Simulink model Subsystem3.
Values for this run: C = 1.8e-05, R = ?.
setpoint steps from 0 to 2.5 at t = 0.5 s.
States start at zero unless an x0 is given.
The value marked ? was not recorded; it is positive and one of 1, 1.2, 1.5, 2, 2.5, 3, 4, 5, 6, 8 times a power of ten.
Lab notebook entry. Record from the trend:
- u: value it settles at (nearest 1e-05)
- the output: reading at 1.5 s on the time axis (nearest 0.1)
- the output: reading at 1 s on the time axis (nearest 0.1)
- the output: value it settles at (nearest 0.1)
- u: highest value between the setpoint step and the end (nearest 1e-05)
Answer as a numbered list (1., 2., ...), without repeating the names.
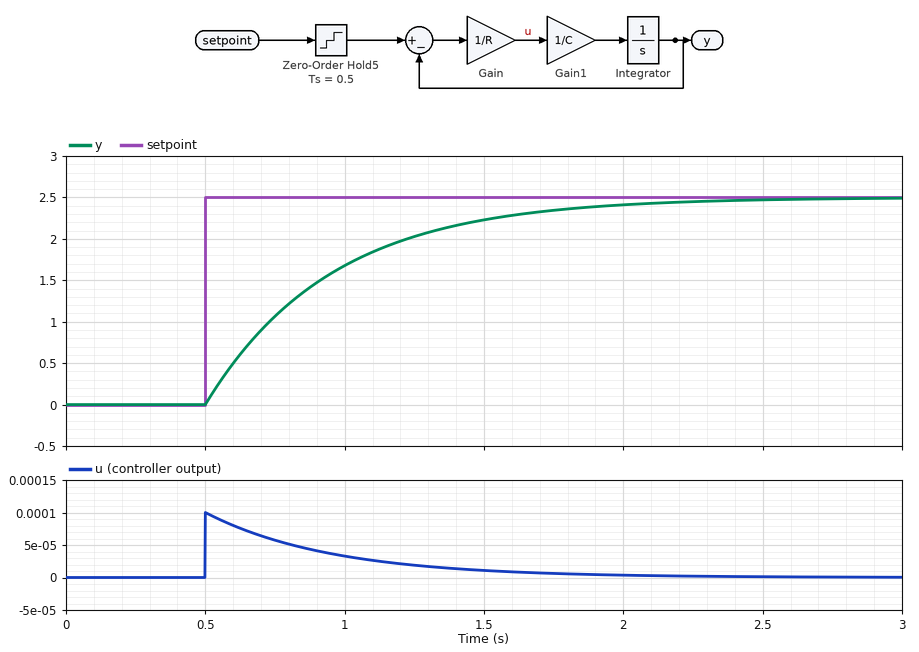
1. 0.00000
2. 2.2
3. 1.7
4. 2.5
5. 0.00010
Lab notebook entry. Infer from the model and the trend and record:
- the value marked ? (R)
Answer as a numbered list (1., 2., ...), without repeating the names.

1. 25000
